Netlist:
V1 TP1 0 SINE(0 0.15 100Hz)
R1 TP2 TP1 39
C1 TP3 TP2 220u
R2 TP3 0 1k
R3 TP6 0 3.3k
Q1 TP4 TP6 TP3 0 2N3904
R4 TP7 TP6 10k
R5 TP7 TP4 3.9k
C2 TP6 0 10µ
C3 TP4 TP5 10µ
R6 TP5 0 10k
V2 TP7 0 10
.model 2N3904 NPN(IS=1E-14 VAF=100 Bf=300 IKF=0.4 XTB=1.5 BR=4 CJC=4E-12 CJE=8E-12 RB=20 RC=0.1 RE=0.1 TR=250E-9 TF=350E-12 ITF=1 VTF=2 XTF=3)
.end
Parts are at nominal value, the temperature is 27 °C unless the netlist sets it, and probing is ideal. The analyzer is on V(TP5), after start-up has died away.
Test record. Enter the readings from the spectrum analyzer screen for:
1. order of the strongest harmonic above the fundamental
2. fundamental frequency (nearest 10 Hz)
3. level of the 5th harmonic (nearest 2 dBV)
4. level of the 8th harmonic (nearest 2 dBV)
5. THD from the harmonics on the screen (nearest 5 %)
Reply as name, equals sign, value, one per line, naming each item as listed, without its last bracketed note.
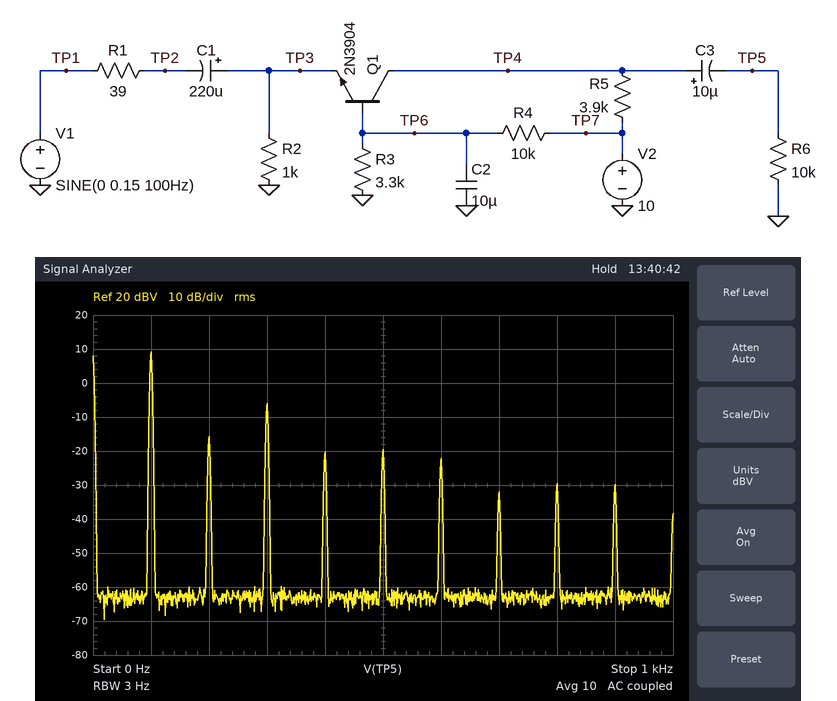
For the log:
order of the strongest harmonic above the fundamental = 3
fundamental frequency = 100 Hz
level of the 5th harmonic = -20 dBV
level of the 8th harmonic = -30 dBV
THD from the harmonics on the screen = 20 %
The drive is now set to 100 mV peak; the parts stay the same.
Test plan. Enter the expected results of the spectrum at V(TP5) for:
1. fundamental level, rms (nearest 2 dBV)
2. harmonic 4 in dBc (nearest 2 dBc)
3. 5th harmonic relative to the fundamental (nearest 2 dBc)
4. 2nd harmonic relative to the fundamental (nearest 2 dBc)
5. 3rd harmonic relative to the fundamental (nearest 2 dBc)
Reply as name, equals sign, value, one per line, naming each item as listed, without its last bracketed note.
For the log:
fundamental level, rms = 8 dBV
harmonic 4 in dBc = -32 dBc
5th harmonic relative to the fundamental = -32 dBc
2nd harmonic relative to the fundamental = -18 dBc
3rd harmonic relative to the fundamental = -18 dBc
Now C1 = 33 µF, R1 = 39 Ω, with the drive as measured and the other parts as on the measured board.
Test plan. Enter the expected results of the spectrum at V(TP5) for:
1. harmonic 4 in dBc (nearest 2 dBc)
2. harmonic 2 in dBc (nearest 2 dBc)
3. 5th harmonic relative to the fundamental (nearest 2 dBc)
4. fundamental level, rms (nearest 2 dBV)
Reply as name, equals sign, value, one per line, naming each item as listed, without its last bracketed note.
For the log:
harmonic 4 in dBc = -32 dBc
harmonic 2 in dBc = -18 dBc
5th harmonic relative to the fundamental = -30 dBc
fundamental level, rms = 8 dBV
